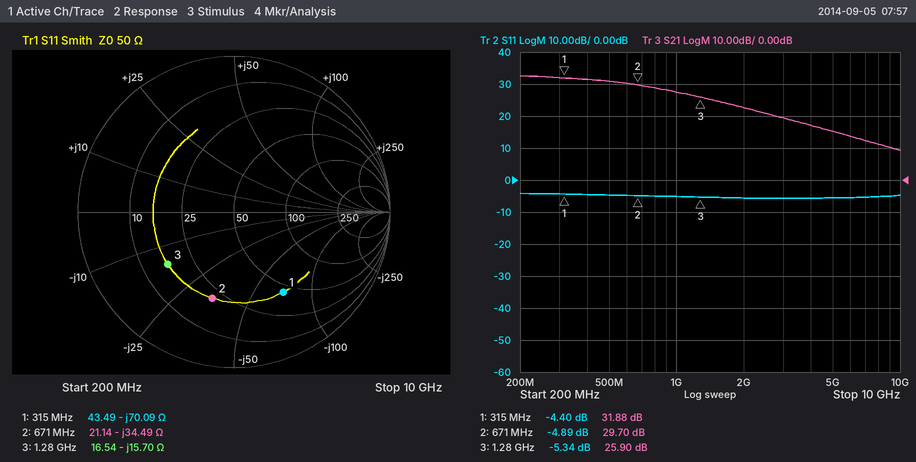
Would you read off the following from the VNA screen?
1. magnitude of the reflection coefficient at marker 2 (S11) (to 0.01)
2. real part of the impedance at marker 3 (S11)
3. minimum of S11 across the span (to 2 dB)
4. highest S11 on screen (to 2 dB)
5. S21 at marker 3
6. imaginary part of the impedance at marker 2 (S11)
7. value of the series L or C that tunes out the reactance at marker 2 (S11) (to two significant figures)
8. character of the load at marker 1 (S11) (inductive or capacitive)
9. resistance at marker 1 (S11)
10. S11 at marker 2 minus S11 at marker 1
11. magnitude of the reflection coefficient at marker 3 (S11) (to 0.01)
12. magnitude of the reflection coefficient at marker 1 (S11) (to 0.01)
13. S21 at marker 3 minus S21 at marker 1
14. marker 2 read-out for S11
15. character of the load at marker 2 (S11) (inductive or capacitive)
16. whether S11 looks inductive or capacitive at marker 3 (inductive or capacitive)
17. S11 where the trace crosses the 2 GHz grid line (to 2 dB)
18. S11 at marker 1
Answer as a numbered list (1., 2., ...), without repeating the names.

1. 0.57
2. 16.54 Ω
3. -6 dB
4. -4 dB
5. 25.90 dB
6. -34.49 Ω
7. 8.2 nH
8. capacitive
9. 43.49 Ω
10. -0.49 dB
11. 0.54
12. 0.60
13. -5.98 dB
14. -4.89 dB
15. capacitive
16. capacitive
17. -6 dB
18. -4.40 dB
